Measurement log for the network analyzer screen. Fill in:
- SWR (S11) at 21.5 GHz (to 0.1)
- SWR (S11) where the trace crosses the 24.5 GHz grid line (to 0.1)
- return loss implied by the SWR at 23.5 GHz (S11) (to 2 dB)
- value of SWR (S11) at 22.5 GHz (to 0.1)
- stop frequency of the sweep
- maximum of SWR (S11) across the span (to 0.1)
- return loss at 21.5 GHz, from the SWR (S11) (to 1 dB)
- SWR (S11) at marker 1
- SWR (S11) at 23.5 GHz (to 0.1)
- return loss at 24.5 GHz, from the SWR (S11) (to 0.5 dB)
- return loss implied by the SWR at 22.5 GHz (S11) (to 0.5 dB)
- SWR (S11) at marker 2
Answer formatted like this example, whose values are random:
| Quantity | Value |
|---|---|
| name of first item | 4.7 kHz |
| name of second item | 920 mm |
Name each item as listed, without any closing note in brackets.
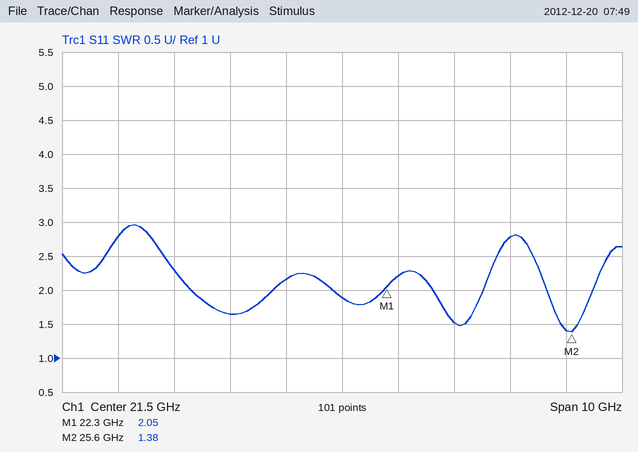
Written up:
| Quantity | Value |
|---|---|
| SWR (S11) at 21.5 GHz | 1.9 |
| SWR (S11) where the trace crosses the 24.5 GHz grid line | 2.8 |
| return loss implied by the SWR at 23.5 GHz (S11) | 14 dB |
| value of SWR (S11) at 22.5 GHz | 2.2 |
| stop frequency of the sweep | 26.5 GHz |
| maximum of SWR (S11) across the span | 3.0 |
| return loss at 21.5 GHz, from the SWR (S11) | 10 dB |
| SWR (S11) at marker 1 | 2.05 |
| SWR (S11) at 23.5 GHz | 1.5 |
| return loss at 24.5 GHz, from the SWR (S11) | 6.5 dB |
| return loss implied by the SWR at 22.5 GHz (S11) | 8.5 dB |
| SWR (S11) at marker 2 | 1.38 |
